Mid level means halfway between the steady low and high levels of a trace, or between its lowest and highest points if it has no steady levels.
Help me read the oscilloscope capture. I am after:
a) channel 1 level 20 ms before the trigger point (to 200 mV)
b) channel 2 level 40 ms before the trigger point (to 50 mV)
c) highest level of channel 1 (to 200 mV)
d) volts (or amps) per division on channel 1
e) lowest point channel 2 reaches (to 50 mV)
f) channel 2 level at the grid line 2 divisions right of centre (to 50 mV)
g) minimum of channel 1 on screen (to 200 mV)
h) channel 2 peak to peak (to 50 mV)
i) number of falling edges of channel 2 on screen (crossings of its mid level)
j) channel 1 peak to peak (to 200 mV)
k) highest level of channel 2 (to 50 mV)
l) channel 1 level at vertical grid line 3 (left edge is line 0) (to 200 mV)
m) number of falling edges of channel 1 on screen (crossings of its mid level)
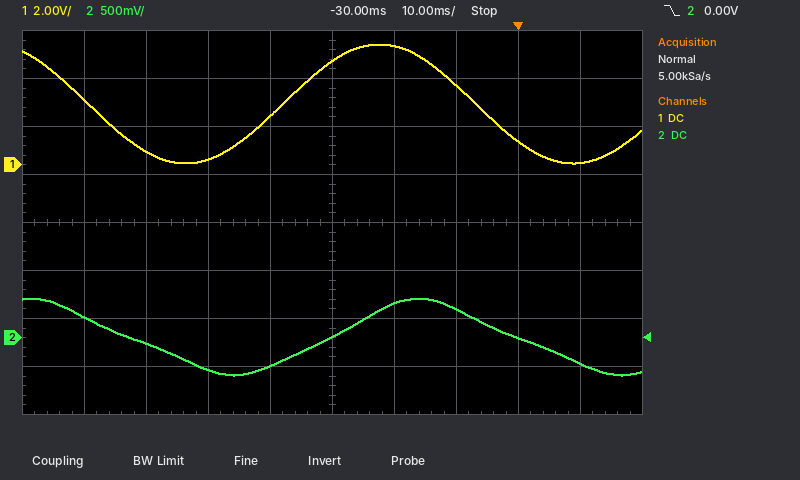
5.0 V
-300 mV
5.0 V
2 V
-400 mV
300 mV
0.0 V
800 mV
2
5.0 V
400 mV
200 mV
2
